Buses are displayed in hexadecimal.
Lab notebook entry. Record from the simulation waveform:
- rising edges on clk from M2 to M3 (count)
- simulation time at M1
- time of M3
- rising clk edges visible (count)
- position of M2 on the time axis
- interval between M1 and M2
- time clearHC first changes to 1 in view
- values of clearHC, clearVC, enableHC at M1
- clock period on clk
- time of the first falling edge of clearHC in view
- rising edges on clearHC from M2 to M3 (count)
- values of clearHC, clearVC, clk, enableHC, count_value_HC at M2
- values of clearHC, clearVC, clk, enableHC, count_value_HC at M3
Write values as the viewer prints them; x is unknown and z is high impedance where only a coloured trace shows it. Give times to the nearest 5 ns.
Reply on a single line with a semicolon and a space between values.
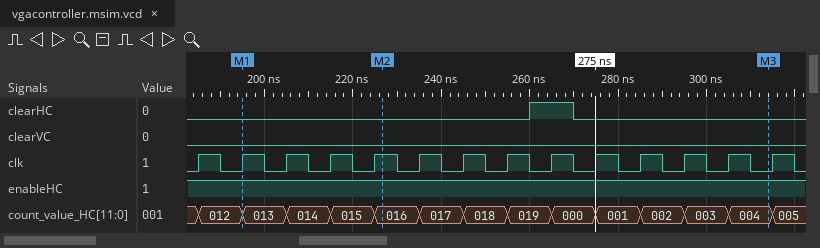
8; 195 ns; 315 ns; 14; 225 ns; 30 ns; 260 ns; clearHC=0, clearVC=0, enableHC=1; 10 ns; 270 ns; 1; clearHC=0, clearVC=0, clk=1, enableHC=1, count_value_HC=016; clearHC=0, clearVC=0, clk=0, enableHC=1, count_value_HC=004
